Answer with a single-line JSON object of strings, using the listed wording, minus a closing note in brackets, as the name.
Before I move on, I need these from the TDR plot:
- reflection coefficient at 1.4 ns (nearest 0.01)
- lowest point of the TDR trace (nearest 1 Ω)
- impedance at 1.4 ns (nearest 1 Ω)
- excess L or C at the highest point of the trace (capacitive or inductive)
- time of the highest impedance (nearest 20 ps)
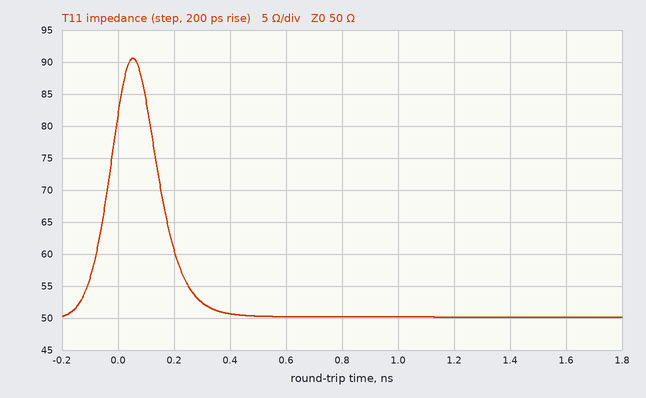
{"reflection coefficient at 1.4 ns": "0.00", "lowest point of the TDR trace": "50 Ω", "impedance at 1.4 ns": "50 Ω", "excess L or C at the highest point of the trace": "inductive", "time of the highest impedance": "60 ps"}
